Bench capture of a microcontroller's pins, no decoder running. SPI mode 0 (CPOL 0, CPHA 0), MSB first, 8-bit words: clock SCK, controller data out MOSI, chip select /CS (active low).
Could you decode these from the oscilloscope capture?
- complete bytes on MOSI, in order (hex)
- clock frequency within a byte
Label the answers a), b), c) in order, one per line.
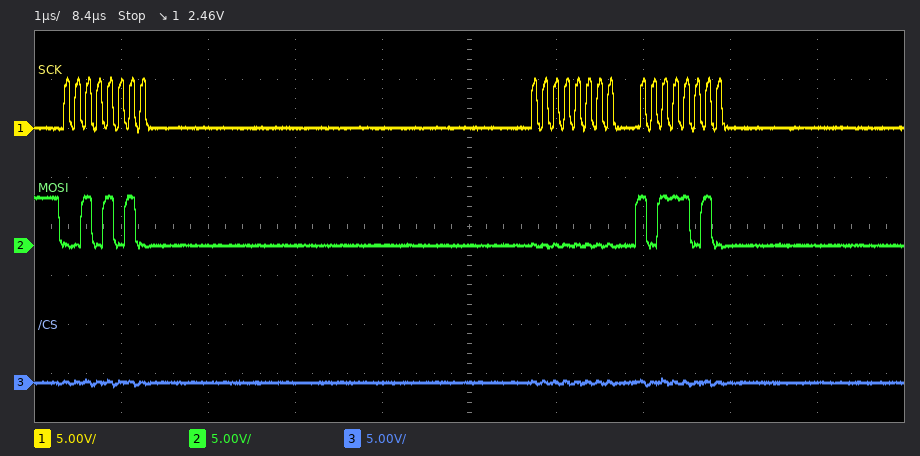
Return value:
a) 2A 00 BA
b) 8 MHz
